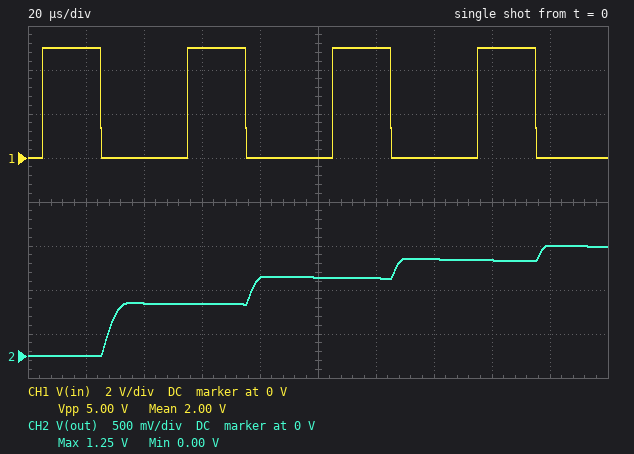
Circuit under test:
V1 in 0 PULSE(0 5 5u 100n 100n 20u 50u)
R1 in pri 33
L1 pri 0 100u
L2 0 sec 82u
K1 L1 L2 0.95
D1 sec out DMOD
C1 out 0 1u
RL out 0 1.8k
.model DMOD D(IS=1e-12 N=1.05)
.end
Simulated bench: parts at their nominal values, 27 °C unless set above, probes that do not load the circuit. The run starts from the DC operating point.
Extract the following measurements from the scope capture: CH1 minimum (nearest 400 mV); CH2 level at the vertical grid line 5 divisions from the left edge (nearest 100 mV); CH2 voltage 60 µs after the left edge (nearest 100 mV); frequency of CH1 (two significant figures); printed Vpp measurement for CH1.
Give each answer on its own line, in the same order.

0 V
900 mV
600 mV
20 kHz
5.00 V
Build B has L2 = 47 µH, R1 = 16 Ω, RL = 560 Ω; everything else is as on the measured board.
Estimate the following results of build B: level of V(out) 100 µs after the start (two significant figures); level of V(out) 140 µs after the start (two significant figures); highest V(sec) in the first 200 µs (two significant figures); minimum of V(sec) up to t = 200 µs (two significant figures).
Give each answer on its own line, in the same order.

1.3 V
1.4 V
2.2 V
-3.2 V
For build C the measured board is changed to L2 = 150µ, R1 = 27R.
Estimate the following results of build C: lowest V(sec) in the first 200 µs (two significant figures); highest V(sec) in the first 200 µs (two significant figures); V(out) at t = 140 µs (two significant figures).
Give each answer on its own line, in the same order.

-5.7 V
2.4 V
1.5 V
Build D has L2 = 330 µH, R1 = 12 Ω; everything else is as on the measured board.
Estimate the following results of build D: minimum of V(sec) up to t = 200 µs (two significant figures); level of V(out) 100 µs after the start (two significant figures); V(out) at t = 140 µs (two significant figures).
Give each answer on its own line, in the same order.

-8.6 V
2.8 V
3.2 V
